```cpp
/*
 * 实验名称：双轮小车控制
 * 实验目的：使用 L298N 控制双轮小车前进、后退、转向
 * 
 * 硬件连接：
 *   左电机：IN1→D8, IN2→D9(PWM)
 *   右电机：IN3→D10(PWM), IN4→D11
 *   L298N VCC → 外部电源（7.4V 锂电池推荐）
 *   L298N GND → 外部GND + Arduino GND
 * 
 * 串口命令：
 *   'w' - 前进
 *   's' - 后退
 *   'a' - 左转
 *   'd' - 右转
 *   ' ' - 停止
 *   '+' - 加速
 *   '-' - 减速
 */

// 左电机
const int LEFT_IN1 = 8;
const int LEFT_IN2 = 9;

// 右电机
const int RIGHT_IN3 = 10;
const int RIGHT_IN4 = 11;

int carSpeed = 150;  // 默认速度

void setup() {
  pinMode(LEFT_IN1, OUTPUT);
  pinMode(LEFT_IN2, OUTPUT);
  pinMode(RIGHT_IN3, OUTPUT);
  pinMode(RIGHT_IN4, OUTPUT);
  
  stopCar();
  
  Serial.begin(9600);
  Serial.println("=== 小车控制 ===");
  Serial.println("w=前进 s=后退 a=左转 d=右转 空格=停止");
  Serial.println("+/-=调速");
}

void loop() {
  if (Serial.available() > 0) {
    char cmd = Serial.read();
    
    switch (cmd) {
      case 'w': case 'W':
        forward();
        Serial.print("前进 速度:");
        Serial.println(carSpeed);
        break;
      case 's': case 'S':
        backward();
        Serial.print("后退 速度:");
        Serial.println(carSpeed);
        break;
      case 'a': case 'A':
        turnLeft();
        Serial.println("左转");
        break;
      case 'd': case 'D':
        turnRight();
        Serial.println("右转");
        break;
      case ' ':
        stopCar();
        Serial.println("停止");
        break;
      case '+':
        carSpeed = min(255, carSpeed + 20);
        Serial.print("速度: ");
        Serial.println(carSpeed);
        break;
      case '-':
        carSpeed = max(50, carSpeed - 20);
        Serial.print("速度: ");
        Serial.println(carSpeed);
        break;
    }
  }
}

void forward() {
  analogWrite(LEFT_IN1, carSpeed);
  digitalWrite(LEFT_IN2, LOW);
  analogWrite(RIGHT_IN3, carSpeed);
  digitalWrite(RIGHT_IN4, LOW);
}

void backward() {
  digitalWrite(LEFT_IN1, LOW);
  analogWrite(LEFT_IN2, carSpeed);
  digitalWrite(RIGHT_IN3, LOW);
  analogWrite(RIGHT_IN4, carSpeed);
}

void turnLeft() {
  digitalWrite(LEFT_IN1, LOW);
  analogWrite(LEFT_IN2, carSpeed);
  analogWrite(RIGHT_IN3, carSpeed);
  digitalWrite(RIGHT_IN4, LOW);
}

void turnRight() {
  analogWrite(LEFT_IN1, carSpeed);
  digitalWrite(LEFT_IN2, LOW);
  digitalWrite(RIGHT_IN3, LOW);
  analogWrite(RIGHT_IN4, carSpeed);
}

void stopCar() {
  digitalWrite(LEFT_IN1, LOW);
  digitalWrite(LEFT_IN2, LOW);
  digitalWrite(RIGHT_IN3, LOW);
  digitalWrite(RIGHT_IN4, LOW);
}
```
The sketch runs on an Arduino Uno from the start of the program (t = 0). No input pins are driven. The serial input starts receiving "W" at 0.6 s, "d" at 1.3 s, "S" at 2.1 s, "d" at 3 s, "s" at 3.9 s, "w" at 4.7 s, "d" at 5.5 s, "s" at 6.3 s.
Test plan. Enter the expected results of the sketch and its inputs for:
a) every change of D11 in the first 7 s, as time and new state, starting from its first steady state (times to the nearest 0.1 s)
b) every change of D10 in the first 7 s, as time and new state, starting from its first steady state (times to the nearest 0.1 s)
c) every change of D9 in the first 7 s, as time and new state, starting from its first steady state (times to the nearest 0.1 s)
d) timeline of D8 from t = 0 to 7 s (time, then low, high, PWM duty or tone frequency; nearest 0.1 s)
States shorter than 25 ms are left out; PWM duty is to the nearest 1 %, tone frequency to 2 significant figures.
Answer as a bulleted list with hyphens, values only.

- 0 s low; 1.3 s PWM 59 %; 4.7 s low; 5.5 s PWM 59 %
- 0 s low; 0.6 s PWM 59 %; 1.3 s low; 4.7 s PWM 59 %; 5.5 s low
- 0 s low; 2.1 s PWM 59 %; 3 s low; 3.9 s PWM 59 %; 4.7 s low; 6.3 s PWM 59 %
- 0 s low; 0.6 s high; 2.1 s low; 3 s high; 3.9 s low; 4.7 s high; 6.3 s low
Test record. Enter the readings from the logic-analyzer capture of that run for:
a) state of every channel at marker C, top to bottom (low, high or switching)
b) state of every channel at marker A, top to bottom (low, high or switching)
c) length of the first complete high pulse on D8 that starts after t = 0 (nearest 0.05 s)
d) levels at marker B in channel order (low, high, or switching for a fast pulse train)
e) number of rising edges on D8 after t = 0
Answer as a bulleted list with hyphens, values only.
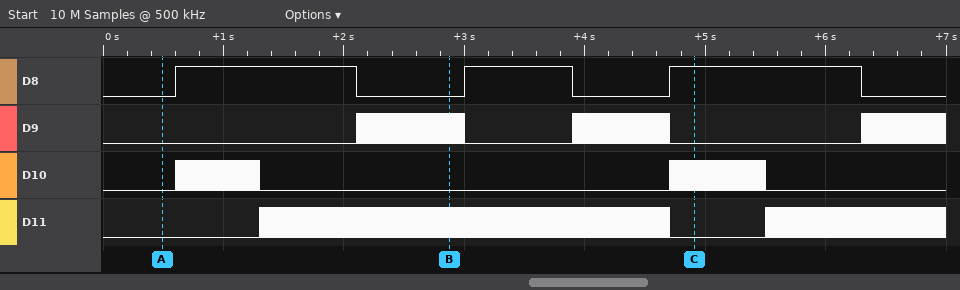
- D8 high, D9 low, D10 switching, D11 low
- D8 low, D9 low, D10 low, D11 low
- 1.50 s
- D8 low, D9 switching, D10 low, D11 switching
- 3
